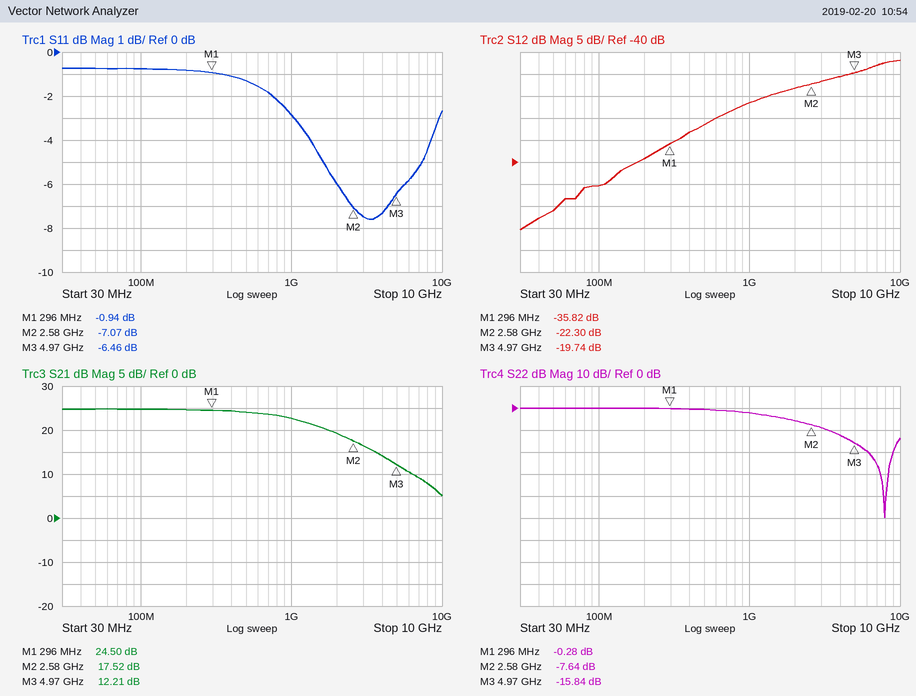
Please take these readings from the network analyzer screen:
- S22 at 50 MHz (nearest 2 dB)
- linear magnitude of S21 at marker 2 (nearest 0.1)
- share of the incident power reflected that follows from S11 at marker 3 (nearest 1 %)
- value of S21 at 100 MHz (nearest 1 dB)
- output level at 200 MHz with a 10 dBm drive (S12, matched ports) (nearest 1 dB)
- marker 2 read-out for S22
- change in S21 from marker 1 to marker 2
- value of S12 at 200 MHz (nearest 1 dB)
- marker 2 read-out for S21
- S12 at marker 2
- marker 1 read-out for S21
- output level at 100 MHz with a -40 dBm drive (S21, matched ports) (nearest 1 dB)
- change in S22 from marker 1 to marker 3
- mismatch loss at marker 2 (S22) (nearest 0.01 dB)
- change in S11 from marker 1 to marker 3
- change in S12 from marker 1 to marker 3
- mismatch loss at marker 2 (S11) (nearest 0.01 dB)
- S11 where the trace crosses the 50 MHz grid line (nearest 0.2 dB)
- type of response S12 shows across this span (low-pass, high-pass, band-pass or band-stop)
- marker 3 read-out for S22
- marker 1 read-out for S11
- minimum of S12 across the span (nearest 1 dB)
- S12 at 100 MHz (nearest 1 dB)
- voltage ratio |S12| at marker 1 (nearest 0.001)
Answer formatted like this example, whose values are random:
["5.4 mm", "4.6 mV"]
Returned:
["0 dB", "7.5", "23 %", "25 dB", "-29 dBm", "-7.64 dB", "-6.98 dB", "-39 dB", "17.52 dB", "-22.30 dB", "24.50 dB", "-15 dBm", "-15.56 dB", "0.82 dB", "-5.52 dB", "16.08 dB", "0.95 dB", "-0.8 dB", "high-pass", "-15.84 dB", "-0.94 dB", "-55 dB", "-45 dB", "0.016"]
